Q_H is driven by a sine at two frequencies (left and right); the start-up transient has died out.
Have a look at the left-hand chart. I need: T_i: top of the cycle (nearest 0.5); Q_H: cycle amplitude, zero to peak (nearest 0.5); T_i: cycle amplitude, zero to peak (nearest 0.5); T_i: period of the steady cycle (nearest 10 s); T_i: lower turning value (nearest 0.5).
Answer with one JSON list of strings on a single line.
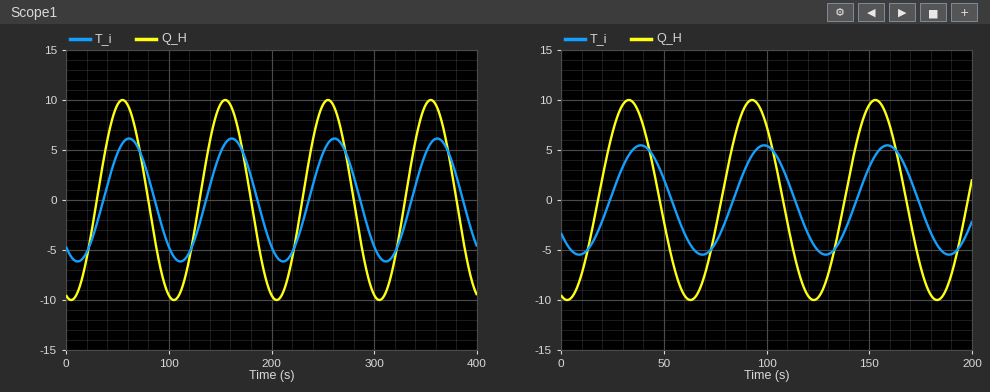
["6.0", "10.0", "6.0", "100 s", "-6.0"]
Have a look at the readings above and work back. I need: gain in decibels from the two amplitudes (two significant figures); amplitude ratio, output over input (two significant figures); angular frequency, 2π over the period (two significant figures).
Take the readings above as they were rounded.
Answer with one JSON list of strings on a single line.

["-4.4 dB", "0.60", "0.063 rad/s"]
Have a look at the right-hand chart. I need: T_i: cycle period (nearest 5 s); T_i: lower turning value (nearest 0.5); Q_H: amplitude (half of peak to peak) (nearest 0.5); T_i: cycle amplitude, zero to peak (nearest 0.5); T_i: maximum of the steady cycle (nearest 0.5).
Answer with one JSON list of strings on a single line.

["60 s", "-5.5", "10.0", "5.5", "5.5"]
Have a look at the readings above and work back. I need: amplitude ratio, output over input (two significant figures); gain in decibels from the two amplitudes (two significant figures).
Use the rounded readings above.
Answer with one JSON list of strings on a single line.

["0.55", "-5.2 dB"]
